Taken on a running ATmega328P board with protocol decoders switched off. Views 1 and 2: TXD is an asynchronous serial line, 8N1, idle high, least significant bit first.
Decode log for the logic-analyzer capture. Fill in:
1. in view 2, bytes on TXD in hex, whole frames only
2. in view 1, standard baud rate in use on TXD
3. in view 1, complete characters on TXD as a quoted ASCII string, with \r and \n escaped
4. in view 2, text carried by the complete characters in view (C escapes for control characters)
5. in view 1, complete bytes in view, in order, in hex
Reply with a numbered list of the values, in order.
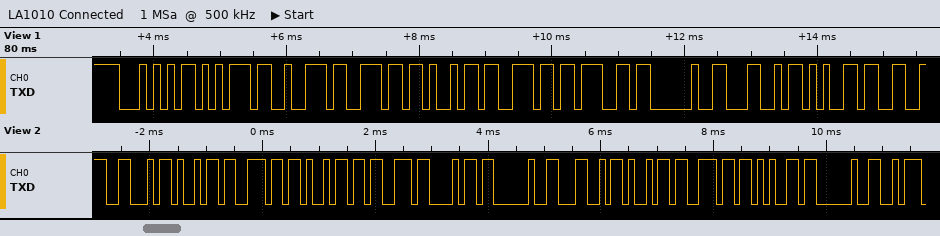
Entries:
1. 0x46 0x69 0x6E 0x69 0x73 0x68 0x20 0x4C 0x69 0x6E 0x65 0x20
2. 9600 baud
3. "Turning Le"
4. "Finish Line "
5. 54 75 72 6E 69 6E 67 20 4C 65
